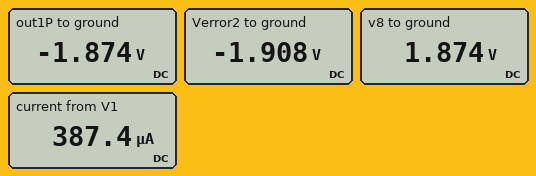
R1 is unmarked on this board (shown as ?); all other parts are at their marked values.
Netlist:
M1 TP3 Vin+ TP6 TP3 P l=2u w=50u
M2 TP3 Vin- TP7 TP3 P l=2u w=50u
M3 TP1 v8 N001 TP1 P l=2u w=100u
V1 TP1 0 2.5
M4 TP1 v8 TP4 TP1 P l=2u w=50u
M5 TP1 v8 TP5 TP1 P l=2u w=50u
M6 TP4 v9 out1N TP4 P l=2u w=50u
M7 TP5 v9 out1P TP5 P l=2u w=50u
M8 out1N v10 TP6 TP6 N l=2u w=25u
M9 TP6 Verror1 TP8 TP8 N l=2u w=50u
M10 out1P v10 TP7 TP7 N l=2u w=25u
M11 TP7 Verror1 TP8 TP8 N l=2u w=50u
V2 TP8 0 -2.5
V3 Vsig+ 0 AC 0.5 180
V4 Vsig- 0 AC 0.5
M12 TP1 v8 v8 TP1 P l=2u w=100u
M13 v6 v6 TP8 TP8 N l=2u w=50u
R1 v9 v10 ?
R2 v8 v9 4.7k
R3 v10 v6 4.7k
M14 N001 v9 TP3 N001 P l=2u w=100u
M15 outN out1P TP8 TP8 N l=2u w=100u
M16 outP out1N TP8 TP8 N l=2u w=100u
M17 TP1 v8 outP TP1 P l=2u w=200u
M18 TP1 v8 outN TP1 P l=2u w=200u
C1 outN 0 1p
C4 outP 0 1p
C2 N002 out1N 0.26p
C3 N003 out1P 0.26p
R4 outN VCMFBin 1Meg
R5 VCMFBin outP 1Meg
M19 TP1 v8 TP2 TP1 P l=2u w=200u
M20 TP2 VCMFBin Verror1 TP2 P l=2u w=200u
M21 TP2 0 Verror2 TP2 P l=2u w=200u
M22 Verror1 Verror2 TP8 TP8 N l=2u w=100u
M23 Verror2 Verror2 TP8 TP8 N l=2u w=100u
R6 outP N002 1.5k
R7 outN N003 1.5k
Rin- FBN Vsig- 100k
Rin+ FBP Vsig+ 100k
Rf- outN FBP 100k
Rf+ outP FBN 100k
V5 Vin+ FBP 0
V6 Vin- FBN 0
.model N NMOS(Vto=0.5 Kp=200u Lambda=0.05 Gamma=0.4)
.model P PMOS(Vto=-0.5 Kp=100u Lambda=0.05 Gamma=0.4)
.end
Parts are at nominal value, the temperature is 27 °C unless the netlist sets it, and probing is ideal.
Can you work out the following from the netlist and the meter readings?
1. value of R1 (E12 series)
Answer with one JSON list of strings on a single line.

["82 kΩ"]
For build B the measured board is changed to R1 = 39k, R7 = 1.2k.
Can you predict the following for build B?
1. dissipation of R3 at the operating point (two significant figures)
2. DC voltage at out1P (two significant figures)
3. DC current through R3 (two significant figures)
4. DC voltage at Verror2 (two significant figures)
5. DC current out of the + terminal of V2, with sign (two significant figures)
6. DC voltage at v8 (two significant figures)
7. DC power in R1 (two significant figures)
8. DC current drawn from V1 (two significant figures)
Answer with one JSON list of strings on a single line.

["27 µW", "-1.8 V", "76 µA", "-1.9 V", "-710 µA", "1.8 V", "220 µW", "710 µA"]
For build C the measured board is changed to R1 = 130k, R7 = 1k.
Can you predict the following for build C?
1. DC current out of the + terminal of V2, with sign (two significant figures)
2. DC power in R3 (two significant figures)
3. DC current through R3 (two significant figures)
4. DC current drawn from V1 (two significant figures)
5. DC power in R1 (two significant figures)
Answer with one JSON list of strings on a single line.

["-260 µA", "3.5 µW", "27 µA", "260 µA", "96 µW"]
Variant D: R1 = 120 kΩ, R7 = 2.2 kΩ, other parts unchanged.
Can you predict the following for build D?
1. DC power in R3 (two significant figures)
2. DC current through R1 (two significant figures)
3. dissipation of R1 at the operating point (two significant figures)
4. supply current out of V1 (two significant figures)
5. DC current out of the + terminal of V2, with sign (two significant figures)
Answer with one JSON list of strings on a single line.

["4.0 µW", "29 µA", "100 µW", "280 µA", "-280 µA"]
